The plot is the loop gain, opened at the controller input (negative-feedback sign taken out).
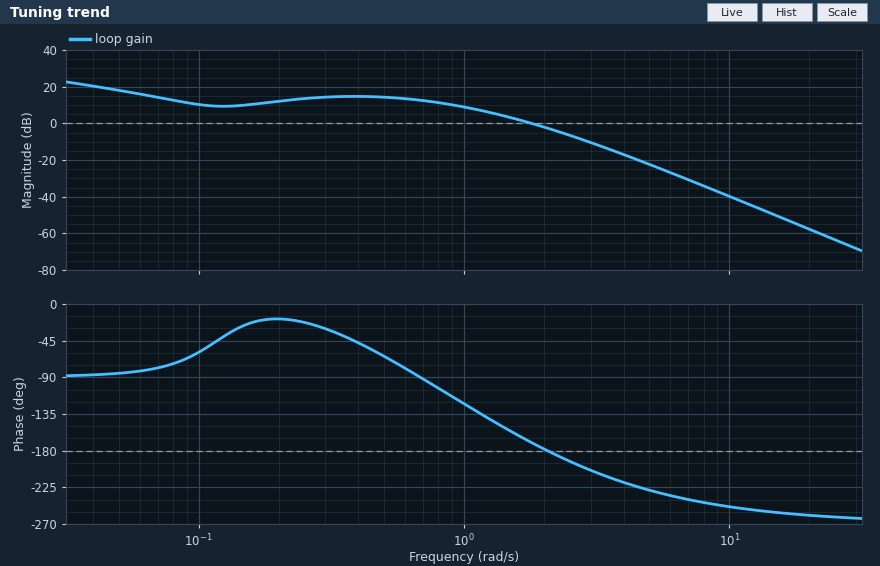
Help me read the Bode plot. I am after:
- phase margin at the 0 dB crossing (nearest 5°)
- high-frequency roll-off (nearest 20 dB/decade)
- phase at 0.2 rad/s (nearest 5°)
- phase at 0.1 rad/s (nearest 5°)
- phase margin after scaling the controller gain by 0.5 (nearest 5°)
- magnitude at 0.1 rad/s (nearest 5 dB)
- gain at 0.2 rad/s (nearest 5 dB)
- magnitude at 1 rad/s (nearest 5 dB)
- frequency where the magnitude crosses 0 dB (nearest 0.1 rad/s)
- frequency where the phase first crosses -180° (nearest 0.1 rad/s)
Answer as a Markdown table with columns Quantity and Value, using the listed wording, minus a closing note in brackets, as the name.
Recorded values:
| Quantity | Value |
|---|---|
| phase margin at the 0 dB crossing | 10° |
| high-frequency roll-off | -60 dB/decade |
| phase at 0.2 rad/s | -20° |
| phase at 0.1 rad/s | -60° |
| phase margin after scaling the controller gain by 0.5 | 40° |
| magnitude at 0.1 rad/s | 10 dB |
| gain at 0.2 rad/s | 10 dB |
| magnitude at 1 rad/s | 10 dB |
| frequency where the magnitude crosses 0 dB | 1.8 rad/s |
| frequency where the phase first crosses -180° | 2.1 rad/s |
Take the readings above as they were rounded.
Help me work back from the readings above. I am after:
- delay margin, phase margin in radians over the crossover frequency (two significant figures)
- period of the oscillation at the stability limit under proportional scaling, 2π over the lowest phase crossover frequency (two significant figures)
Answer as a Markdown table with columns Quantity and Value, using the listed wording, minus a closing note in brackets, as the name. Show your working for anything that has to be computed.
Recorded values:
| Quantity | Value |
|---|---|
| delay margin, phase margin in radians over the crossover frequency | 10 × π / 180 / 1.8 = 0.097 s |
| period of the oscillation at the stability limit under proportional scaling, 2π over the lowest phase crossover frequency | 2π / 2.1 = 3.0 s |
